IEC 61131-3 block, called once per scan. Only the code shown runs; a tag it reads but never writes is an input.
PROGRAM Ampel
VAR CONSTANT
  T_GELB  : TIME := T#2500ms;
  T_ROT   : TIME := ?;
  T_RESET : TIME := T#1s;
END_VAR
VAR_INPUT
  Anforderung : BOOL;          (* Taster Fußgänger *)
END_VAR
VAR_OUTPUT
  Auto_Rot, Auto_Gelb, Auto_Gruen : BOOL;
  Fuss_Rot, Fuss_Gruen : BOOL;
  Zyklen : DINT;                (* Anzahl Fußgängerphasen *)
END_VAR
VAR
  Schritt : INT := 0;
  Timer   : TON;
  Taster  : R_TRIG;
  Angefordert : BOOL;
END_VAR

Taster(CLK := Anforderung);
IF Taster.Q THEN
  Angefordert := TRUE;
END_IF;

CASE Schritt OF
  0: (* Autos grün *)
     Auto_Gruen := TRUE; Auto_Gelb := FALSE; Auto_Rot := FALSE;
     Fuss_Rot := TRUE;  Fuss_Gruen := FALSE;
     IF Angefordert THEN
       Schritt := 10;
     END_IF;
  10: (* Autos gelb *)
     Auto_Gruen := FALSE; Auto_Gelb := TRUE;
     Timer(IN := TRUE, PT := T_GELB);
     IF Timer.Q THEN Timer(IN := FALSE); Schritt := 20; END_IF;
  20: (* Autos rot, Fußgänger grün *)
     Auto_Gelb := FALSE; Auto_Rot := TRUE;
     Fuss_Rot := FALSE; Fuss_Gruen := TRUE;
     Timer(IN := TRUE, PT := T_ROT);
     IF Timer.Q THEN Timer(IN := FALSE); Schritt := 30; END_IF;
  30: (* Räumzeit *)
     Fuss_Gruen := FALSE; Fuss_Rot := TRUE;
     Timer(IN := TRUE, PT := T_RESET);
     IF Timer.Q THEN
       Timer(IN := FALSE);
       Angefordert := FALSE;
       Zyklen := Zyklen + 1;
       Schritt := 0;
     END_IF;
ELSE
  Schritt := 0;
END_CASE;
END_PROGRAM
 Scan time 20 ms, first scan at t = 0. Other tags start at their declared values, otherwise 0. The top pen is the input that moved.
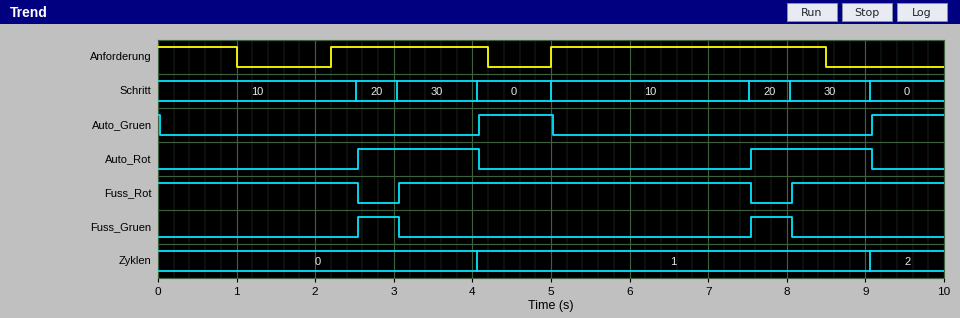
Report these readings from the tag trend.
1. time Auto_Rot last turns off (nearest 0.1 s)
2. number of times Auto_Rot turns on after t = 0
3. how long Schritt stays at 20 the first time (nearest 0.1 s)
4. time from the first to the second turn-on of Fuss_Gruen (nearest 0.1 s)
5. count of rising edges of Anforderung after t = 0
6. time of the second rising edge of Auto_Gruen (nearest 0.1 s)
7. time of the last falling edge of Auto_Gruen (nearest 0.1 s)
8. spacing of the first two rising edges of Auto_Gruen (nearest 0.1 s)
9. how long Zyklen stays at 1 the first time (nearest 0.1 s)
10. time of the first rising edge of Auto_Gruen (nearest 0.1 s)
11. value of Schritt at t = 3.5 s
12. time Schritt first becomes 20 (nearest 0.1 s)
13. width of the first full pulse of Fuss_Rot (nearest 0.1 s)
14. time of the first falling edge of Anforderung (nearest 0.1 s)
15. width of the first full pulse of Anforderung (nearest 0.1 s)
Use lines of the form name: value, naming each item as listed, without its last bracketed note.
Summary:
time Auto_Rot last turns off: 9.1 s
number of times Auto_Rot turns on after t = 0: 2
how long Schritt stays at 20 the first time: 0.5 s
time from the first to the second turn-on of Fuss_Gruen: 5.0 s
count of rising edges of Anforderung after t = 0: 2
time of the second rising edge of Auto_Gruen: 9.1 s
time of the last falling edge of Auto_Gruen: 5.0 s
spacing of the first two rising edges of Auto_Gruen: 5.0 s
how long Zyklen stays at 1 the first time: 5.0 s
time of the first rising edge of Auto_Gruen: 4.1 s
value of Schritt at t = 3.5 s: 30
time Schritt first becomes 20: 2.5 s
width of the first full pulse of Fuss_Rot: 4.5 s
time of the first falling edge of Anforderung: 1.0 s
width of the first full pulse of Anforderung: 2.0 s
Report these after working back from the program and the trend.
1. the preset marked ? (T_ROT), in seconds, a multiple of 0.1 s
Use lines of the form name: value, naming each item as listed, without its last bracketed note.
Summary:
the preset marked ? (T_ROT), in seconds, a multiple of 0.1 s: 0.5 s
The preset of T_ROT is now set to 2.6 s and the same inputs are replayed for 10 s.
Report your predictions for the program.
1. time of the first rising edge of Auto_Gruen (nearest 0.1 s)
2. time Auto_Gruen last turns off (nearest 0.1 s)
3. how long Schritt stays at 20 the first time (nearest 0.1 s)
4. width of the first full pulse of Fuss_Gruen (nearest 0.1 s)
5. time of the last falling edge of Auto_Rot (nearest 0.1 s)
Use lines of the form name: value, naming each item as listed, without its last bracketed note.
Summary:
time of the first rising edge of Auto_Gruen: 6.2 s
time Auto_Gruen last turns off: 0.0 s
how long Schritt stays at 20 the first time: 2.6 s
width of the first full pulse of Fuss_Gruen: 2.6 s
time of the last falling edge of Auto_Rot: 6.2 s
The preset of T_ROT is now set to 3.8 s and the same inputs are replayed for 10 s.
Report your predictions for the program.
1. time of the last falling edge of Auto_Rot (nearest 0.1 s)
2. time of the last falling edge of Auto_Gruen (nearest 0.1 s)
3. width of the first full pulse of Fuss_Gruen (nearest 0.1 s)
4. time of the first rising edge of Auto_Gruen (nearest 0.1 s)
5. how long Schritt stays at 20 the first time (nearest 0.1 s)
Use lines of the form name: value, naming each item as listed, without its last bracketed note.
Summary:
time of the last falling edge of Auto_Rot: 7.4 s
time of the last falling edge of Auto_Gruen: 0.0 s
width of the first full pulse of Fuss_Gruen: 3.8 s
time of the first rising edge of Auto_Gruen: 7.4 s
how long Schritt stays at 20 the first time: 3.8 s
